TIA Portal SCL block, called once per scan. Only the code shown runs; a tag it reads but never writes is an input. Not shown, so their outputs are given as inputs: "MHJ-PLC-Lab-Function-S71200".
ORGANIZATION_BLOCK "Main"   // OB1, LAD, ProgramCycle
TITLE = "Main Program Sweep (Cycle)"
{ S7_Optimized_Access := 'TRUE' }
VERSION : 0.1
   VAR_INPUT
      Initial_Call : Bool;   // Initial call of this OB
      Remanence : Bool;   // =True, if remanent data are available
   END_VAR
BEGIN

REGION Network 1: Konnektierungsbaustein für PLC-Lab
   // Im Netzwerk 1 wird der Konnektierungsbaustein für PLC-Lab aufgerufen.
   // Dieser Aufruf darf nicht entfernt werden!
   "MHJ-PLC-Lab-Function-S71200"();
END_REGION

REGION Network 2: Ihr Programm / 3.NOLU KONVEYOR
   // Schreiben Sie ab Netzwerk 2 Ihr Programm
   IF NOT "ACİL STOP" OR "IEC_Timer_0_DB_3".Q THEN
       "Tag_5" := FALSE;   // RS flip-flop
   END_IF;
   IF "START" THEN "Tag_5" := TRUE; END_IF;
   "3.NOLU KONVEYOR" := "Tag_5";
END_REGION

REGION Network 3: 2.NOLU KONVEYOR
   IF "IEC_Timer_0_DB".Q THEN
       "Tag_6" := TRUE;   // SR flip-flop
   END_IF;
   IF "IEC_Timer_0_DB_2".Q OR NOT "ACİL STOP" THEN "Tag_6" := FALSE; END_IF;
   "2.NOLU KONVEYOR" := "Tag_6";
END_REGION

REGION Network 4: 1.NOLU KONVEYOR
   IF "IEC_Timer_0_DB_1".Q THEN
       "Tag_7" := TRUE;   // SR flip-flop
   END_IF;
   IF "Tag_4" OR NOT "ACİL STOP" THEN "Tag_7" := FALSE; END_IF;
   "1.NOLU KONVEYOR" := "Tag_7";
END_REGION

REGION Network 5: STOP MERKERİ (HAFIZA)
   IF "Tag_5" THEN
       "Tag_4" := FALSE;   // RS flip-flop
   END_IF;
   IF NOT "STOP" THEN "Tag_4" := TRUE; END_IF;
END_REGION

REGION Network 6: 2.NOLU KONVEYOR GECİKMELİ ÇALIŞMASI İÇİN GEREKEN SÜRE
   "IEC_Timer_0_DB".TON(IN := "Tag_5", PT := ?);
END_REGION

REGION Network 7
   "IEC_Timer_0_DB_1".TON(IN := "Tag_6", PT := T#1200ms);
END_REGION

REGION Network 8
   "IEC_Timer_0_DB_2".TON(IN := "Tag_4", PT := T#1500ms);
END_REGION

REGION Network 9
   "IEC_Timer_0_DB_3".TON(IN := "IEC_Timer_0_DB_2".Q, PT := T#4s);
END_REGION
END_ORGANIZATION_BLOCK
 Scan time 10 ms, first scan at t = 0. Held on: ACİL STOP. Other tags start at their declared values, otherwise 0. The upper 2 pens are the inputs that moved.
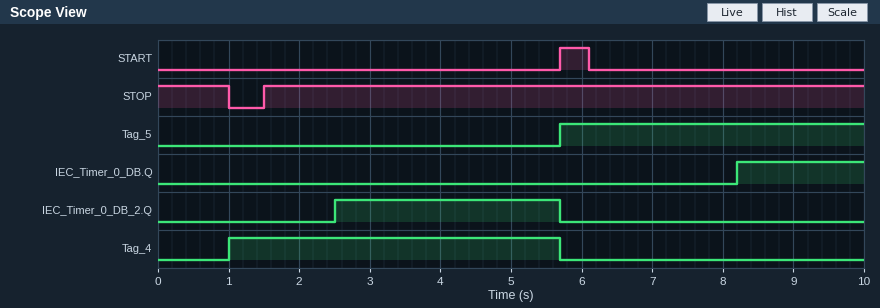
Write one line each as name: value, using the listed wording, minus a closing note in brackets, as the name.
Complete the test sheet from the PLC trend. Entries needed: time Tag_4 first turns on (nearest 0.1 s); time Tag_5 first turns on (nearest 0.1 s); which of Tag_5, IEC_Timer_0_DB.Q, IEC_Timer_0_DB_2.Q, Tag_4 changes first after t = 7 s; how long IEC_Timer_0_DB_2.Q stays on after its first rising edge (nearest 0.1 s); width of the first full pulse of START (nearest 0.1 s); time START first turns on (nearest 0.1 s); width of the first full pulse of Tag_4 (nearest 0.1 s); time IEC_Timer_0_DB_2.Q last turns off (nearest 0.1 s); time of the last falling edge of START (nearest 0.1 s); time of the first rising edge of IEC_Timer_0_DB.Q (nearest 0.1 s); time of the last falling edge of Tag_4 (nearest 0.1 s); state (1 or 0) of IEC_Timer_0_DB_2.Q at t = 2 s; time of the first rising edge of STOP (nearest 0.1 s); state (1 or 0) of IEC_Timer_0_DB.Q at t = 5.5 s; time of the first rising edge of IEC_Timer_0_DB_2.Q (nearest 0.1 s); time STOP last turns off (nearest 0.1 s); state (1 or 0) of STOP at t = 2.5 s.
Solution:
time Tag_4 first turns on: 1.0 s
time Tag_5 first turns on: 5.7 s
which of Tag_5, IEC_Timer_0_DB.Q, IEC_Timer_0_DB_2.Q, Tag_4 changes first after t = 7 s: IEC_Timer_0_DB.Q
how long IEC_Timer_0_DB_2.Q stays on after its first rising edge: 3.2 s
width of the first full pulse of START: 0.4 s
time START first turns on: 5.7 s
width of the first full pulse of Tag_4: 4.7 s
time IEC_Timer_0_DB_2.Q last turns off: 5.7 s
time of the last falling edge of START: 6.1 s
time of the first rising edge of IEC_Timer_0_DB.Q: 8.2 s
time of the last falling edge of Tag_4: 5.7 s
state (1 or 0) of IEC_Timer_0_DB_2.Q at t = 2 s: 0
time of the first rising edge of STOP: 1.5 s
state (1 or 0) of IEC_Timer_0_DB.Q at t = 5.5 s: 0
time of the first rising edge of IEC_Timer_0_DB_2.Q: 2.5 s
time STOP last turns off: 1.0 s
state (1 or 0) of STOP at t = 2.5 s: 1
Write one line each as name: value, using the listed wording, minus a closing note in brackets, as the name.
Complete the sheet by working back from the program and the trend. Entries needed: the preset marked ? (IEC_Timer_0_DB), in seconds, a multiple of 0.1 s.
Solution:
the preset marked ? (IEC_Timer_0_DB), in seconds, a multiple of 0.1 s: 2.5 s
